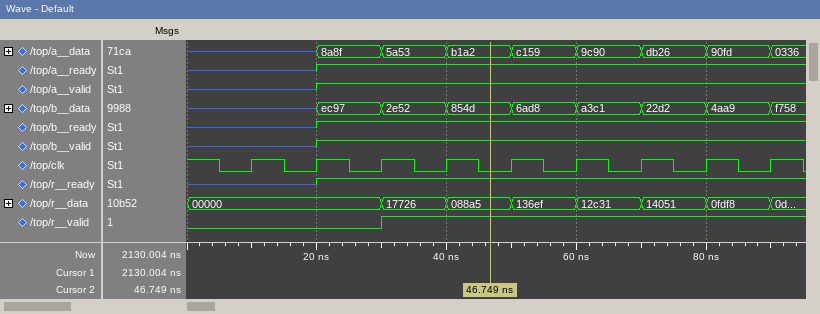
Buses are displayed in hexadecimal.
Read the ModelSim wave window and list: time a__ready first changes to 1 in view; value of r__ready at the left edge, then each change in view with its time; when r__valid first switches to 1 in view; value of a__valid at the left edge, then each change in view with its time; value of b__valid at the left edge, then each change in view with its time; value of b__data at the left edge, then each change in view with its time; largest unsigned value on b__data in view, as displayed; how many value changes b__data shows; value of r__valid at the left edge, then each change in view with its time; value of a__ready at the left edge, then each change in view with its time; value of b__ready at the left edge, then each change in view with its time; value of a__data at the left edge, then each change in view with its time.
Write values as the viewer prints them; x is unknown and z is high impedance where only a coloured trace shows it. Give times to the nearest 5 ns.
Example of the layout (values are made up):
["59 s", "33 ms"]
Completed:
["20 ns", "z, 1 at 20 ns", "30 ns", "z, 1 at 20 ns", "z, 1 at 20 ns", "z, ec97 at 20 ns, 2e52 at 30 ns, 854d at 40 ns, 6ad8 at 50 ns, a3c1 at 60 ns, 22d2 at 70 ns, 4aa9 at 80 ns, f758 at 90 ns", "f758", "8", "0, 1 at 30 ns", "z, 1 at 20 ns", "z, 1 at 20 ns", "z, 8a8f at 20 ns, 5a53 at 30 ns, b1a2 at 40 ns, c159 at 50 ns, 9c90 at 60 ns, db26 at 70 ns, 90fd at 80 ns, 0336 at 90 ns"]
